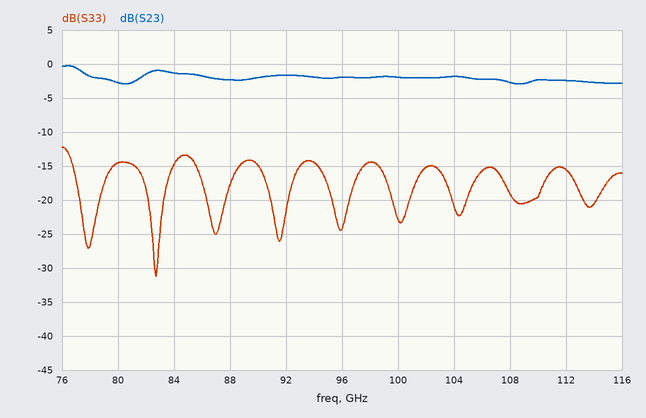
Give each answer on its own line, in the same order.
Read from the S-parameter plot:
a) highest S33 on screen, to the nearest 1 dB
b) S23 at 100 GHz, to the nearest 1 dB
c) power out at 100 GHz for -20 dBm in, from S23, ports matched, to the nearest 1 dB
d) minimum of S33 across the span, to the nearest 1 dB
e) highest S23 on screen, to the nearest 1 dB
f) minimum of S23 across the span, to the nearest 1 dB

-12 dB
-2 dB
-22 dBm
-31 dB
0 dB
-3 dB
